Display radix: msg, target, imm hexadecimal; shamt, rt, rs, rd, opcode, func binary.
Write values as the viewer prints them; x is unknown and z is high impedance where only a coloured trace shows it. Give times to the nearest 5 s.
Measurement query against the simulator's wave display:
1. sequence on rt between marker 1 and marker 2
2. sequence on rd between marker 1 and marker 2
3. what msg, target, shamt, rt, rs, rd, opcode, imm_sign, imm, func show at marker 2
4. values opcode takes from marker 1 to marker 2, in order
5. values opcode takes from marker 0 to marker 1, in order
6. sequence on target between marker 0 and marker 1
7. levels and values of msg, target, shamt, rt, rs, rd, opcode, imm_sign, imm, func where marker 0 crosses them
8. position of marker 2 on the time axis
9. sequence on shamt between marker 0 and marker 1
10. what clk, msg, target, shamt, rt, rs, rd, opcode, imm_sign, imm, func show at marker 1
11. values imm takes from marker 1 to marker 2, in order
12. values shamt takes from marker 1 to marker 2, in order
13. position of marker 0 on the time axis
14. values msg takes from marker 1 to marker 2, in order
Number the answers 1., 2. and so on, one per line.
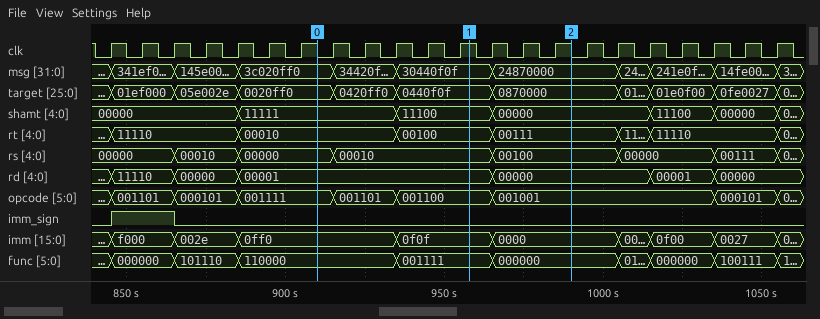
1. 00100, 00111
2. 00001, 00000
3. msg=24870000, target=0870000, shamt=00000, rt=00111, rs=00100, rd=00000, opcode=001001, imm_sign=0, imm=0000, func=000000
4. 001100, 001001
5. 001111, 001101, 001100
6. 0020ff0, 0420ff0, 0440f0f
7. msg=3c020ff0, target=0020ff0, shamt=11111, rt=00010, rs=00000, rd=00001, opcode=001111, imm_sign=0, imm=0ff0, func=110000
8. 990 s
9. 11111, 11100
10. clk=1, msg=30440f0f, target=0440f0f, shamt=11100, rt=00100, rs=00010, rd=00001, opcode=001100, imm_sign=0, imm=0f0f, func=001111
11. 0f0f, 0000
12. 11100, 00000
13. 910 s
14. 30440f0f, 24870000
